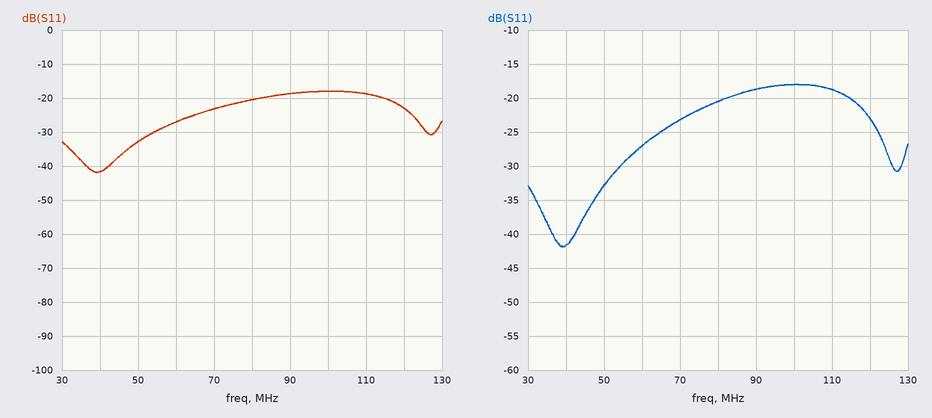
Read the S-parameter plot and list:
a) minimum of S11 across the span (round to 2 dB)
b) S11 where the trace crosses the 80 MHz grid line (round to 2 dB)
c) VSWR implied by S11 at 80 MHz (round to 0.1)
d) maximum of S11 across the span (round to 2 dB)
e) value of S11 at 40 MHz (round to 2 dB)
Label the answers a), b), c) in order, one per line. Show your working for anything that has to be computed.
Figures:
a) -42 dB
b) -20 dB
c) |Γ| = 10^(-20/20) = 0.1000; VSWR = (1 + 0.1000)/(1 − 0.1000) ≈ 1.2
d) -18 dB
e) -42 dB
